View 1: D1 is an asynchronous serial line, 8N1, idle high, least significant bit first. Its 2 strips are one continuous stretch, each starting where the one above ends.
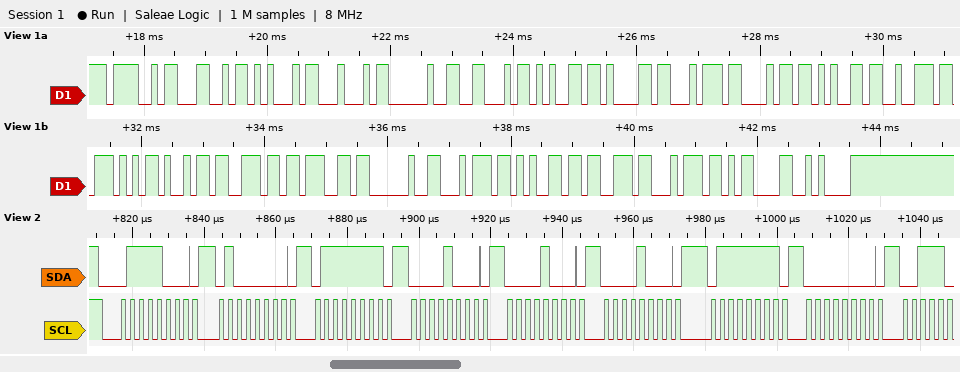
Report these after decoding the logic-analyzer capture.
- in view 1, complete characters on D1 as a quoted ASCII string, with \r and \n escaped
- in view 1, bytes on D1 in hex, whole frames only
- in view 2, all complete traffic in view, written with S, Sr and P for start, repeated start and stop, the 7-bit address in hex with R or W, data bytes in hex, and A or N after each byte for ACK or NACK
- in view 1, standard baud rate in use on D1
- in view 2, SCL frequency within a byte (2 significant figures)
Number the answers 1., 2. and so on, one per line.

1. "OLED FeatherWing test\r\n"
2. 4F 4C 45 44 20 46 65 61 74 68 65 72 57 69 6E 67 20 74 65 73 74 0D 0A
3. S 3CW A 40 A 7F A 08 A 08 A 08 A 7F A 00 A
4. 9600 baud
5. 400 kHz
